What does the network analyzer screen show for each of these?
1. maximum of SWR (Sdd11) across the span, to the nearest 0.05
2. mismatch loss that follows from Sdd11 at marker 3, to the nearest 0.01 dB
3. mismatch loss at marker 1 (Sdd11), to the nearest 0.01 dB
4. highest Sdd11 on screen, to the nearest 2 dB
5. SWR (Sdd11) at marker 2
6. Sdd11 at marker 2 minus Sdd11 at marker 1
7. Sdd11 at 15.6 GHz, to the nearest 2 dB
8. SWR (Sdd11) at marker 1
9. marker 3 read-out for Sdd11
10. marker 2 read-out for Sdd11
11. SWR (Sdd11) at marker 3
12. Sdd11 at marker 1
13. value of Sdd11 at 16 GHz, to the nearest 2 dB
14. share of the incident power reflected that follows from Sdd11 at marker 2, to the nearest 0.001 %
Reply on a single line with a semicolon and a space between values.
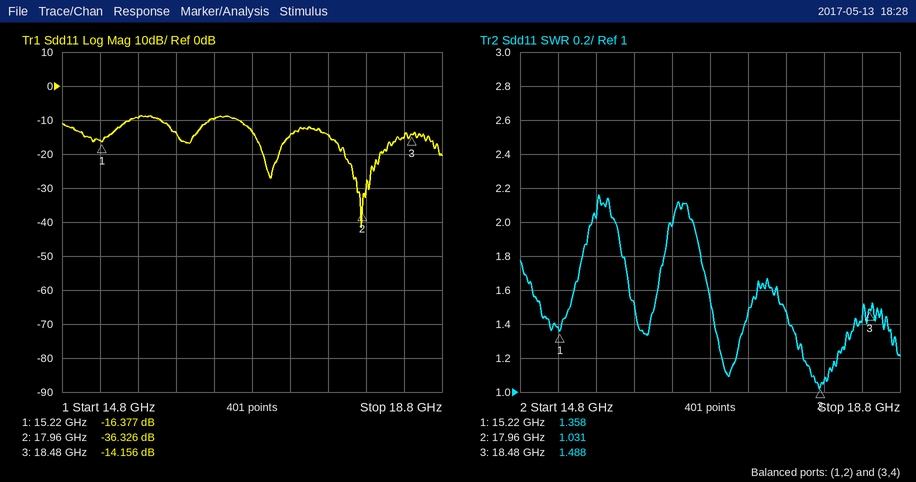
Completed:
2.15; 0.17 dB; 0.10 dB; -8 dB; 1.031; -19.949 dB; -10 dB; 1.358; -14.156 dB; -36.326 dB; 1.488; -16.377 dB; -14 dB; 0.023 %
